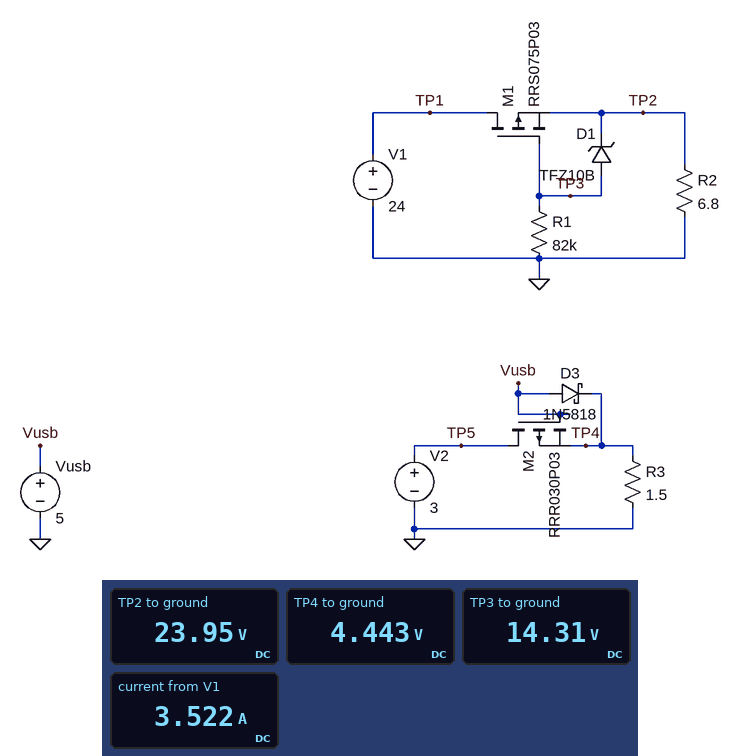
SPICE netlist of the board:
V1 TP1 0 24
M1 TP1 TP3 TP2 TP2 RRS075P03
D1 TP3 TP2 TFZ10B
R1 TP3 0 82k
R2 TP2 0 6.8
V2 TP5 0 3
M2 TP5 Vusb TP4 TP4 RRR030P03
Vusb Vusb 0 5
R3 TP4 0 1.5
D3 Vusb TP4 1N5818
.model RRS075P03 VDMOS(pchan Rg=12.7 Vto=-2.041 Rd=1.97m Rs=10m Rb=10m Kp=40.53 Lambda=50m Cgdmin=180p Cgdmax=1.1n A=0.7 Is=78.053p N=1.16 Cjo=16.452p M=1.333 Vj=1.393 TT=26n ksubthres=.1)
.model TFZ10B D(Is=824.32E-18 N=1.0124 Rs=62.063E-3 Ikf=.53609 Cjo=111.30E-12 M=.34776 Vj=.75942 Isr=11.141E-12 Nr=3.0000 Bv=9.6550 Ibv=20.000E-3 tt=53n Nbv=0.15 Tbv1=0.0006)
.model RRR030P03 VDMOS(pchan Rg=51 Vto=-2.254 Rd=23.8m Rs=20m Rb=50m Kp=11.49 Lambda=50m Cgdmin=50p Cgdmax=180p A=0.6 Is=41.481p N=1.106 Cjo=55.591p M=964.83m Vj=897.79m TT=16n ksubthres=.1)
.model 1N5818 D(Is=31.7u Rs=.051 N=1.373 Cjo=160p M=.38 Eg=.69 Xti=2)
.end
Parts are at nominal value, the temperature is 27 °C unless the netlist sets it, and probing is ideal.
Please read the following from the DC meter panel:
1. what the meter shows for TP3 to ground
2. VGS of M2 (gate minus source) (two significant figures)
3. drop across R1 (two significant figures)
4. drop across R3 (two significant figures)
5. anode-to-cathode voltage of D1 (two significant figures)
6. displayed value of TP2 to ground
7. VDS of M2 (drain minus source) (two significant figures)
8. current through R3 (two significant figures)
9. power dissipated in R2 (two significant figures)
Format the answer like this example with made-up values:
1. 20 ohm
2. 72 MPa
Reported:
1. 14.31 V
2. 560 mV
3. 14 V
4. 4.4 V
5. -9.6 V
6. 23.95 V
7. -1.4 V
8. 3.0 A
9. 84 W
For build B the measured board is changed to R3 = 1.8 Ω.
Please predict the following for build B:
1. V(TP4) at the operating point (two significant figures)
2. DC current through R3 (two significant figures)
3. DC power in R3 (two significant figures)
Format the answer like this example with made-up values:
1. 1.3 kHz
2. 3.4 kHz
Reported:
1. 4.5 V
2. 2.5 A
3. 11 W
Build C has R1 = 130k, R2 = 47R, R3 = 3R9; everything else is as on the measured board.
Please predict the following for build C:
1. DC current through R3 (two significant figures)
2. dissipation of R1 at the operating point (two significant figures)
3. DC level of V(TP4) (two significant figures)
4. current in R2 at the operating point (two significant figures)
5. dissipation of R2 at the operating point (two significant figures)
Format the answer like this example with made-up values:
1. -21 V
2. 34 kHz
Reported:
1. 1.2 A
2. 1.6 mW
3. 4.6 V
4. 510 mA
5. 12 W
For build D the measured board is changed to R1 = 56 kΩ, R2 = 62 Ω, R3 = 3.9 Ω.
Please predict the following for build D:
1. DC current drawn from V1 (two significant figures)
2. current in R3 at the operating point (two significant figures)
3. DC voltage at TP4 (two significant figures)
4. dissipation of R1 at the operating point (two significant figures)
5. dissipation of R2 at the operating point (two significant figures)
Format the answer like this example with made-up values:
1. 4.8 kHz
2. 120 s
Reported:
1. 390 mA
2. 1.2 A
3. 4.6 V
4. 3.7 mW
5. 9.3 W
